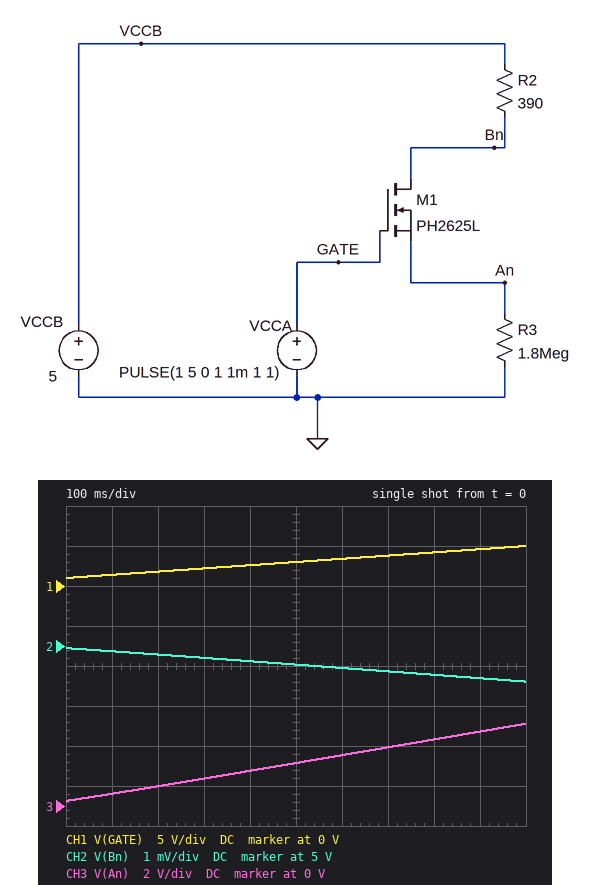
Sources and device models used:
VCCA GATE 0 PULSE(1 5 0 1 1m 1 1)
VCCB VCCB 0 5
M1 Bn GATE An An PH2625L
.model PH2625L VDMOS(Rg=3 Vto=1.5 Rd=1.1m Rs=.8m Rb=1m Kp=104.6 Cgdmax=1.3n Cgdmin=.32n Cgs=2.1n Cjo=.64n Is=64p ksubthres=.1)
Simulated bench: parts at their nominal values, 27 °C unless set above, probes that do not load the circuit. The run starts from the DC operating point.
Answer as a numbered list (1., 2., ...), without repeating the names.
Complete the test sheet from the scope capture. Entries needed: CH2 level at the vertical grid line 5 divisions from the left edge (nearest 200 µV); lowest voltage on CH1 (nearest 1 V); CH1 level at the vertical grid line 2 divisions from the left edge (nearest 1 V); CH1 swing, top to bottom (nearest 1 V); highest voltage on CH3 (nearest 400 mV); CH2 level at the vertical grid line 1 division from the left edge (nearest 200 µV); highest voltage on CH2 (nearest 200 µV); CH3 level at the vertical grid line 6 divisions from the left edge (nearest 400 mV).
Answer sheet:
1. 4.9996 V
2. 1 V
3. 2 V
4. 4 V
5. 4.0 V
6. 4.9998 V
7. 5.0000 V
8. 2.4 V
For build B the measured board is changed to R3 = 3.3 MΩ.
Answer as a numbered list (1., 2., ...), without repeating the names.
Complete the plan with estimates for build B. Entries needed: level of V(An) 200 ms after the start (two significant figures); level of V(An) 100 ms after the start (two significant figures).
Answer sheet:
1. 1.0 V
2. 640 mV
